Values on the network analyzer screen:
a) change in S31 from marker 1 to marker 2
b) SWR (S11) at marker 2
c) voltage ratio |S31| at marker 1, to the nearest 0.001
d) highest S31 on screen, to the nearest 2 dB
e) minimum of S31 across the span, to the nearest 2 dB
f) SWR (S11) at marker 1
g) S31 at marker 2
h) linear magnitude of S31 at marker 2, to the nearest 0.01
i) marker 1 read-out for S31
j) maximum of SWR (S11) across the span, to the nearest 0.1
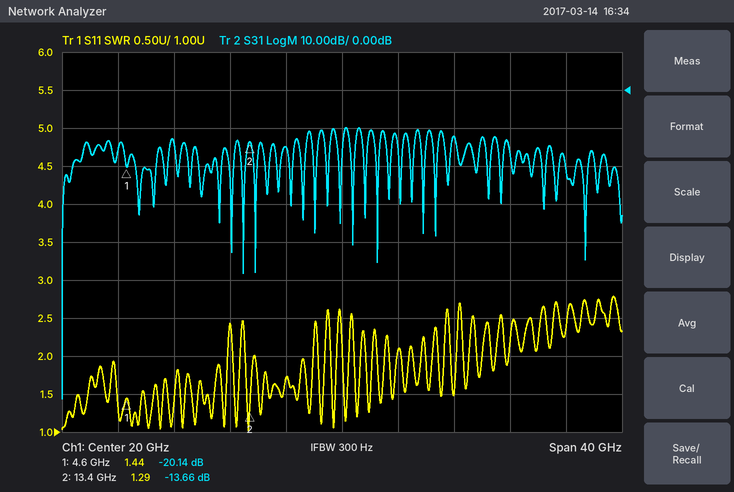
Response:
6.48 dB
1.29
0.098
-10 dB
-82 dB
1.44
-13.66 dB
0.21
-20.14 dB
2.8
